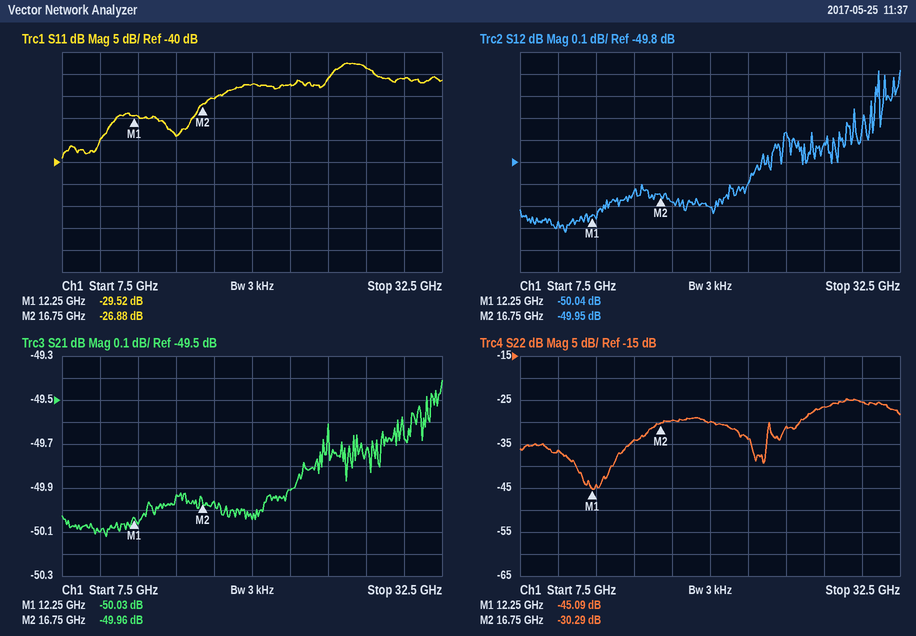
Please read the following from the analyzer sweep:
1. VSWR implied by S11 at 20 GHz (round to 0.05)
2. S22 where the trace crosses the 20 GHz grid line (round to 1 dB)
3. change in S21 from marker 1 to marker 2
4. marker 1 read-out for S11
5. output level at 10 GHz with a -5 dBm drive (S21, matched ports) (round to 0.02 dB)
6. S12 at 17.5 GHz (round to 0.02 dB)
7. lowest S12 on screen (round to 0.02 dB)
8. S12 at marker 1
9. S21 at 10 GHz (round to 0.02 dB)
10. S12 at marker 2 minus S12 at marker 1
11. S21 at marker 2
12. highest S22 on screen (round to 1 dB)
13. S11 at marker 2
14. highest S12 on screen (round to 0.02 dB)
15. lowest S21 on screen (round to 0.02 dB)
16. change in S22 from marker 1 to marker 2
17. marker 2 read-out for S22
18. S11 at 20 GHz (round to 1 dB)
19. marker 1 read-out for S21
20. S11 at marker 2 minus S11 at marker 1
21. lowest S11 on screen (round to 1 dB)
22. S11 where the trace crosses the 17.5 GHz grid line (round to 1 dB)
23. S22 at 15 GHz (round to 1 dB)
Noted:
1.15
-30 dB
0.07 dB
-29.52 dB
-55.10 dBm
-49.98 dB
-50.12 dB
-50.04 dB
-50.10 dB
0.09 dB
-49.96 dB
-25 dB
-26.88 dB
-49.38 dB
-50.12 dB
14.80 dB
-30.29 dB
-22 dB
-50.03 dB
2.64 dB
-39 dB
-26 dB
-34 dB
